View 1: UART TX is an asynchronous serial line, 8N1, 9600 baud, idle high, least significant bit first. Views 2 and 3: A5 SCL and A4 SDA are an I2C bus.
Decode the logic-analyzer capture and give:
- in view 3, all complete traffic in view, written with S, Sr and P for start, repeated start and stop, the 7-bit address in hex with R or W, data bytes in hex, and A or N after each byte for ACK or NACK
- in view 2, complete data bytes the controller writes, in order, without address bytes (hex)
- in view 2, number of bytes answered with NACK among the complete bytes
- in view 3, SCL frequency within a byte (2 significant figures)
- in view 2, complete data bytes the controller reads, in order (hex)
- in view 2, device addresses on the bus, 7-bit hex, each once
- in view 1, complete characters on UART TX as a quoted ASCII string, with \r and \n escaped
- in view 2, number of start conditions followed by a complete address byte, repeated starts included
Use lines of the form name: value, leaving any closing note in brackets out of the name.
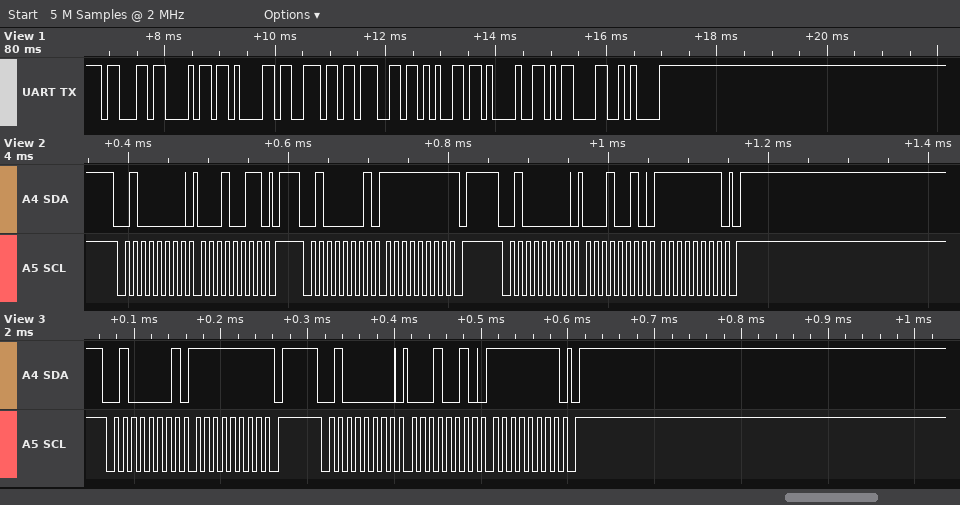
in view 3, all complete traffic in view, written with S, Sr and P for start, repeated start and stop, the 7-bit address in hex with R or W, data bytes in hex, and A or N after each byte for ACK or NACK: S 20R A FF N P S 20W A 12 A FF A P
in view 2, complete data bytes the controller writes, in order, without address bytes: 13 12 FF
in view 2, number of bytes answered with NACK among the complete bytes: 1
in view 3, SCL frequency within a byte: 100 kHz
in view 2, complete data bytes the controller reads, in order: FF
in view 2, device addresses on the bus, 7-bit hex, each once: 0x20
in view 1, complete characters on UART TX as a quoted ASCII string, with \r and \n escaped: "change!\r\n"
in view 2, number of start conditions followed by a complete address byte, repeated starts included: 3
